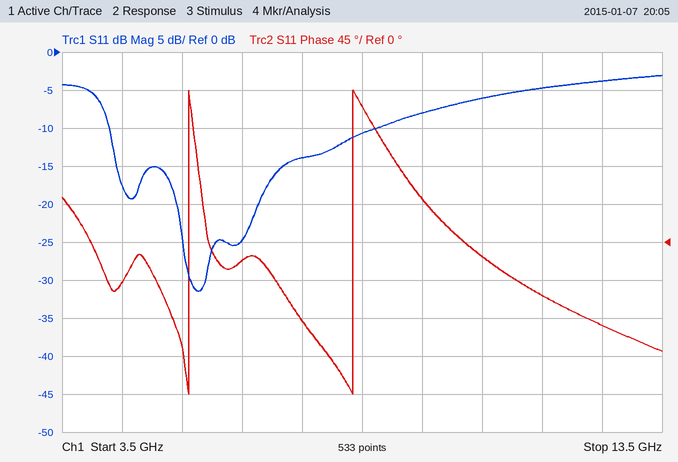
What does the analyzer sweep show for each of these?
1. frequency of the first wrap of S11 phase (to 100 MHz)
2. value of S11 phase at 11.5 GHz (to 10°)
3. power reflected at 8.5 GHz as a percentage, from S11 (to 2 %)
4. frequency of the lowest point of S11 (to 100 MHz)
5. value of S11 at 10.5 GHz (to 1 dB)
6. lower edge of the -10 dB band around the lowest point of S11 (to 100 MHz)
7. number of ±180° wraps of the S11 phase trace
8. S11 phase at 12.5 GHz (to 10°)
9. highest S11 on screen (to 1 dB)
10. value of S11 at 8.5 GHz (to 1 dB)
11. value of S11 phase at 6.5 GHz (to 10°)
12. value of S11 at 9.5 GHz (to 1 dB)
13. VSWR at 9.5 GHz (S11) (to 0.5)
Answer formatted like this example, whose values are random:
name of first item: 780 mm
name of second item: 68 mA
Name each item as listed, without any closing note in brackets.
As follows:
frequency of the first wrap of S11 phase: 5.6 GHz
value of S11 phase at 11.5 GHz: -60°
power reflected at 8.5 GHz as a percentage, from S11: 8 %
frequency of the lowest point of S11: 5.8 GHz
value of S11 at 10.5 GHz: -6 dB
lower edge of the -10 dB band around the lowest point of S11: 4.3 GHz
number of ±180° wraps of the S11 phase trace: 2
S11 phase at 12.5 GHz: -100°
highest S11 on screen: -3 dB
value of S11 at 8.5 GHz: -11 dB
value of S11 phase at 6.5 GHz: -20°
value of S11 at 9.5 GHz: -8 dB
VSWR at 9.5 GHz (S11): 2.5
